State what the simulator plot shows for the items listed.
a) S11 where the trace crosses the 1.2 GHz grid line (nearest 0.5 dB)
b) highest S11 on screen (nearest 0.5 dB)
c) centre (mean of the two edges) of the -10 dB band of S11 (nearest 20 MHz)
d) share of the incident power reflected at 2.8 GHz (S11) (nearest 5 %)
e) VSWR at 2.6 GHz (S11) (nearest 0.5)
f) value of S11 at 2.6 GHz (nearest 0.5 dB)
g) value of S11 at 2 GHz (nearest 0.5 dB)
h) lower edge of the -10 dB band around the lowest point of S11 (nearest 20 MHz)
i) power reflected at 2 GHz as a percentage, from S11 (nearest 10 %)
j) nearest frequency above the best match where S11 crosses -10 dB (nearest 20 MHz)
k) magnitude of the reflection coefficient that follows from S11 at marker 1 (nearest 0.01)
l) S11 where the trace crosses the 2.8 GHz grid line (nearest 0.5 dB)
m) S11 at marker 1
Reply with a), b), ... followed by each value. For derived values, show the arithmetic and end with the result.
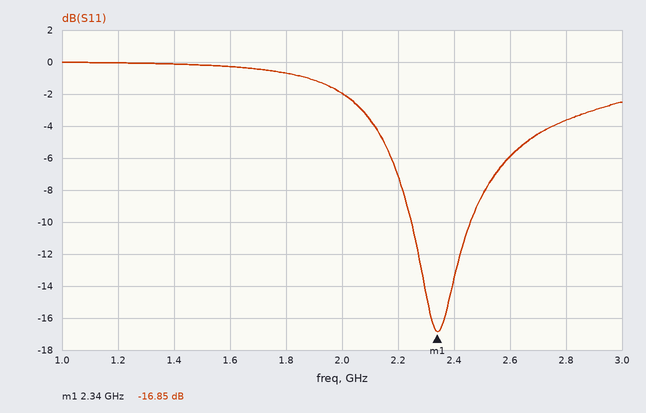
a) 0.0 dB
b) 0.0 dB
c) 2.36 GHz
d) 10^(-3.5/10) ≈ 45 %
e) |Γ| = 10^(-6/20) = 0.5012; VSWR = (1 + 0.5012)/(1 − 0.5012) ≈ 3.0
f) -6.0 dB
g) -2.0 dB
h) 2.24 GHz
i) 10^(-2/10) ≈ 63.1 %, so 60 % to the nearest 10 %
j) 2.46 GHz
k) 10^(-16.85/20) ≈ 0.14
l) -3.5 dB
m) -16.85 dB
